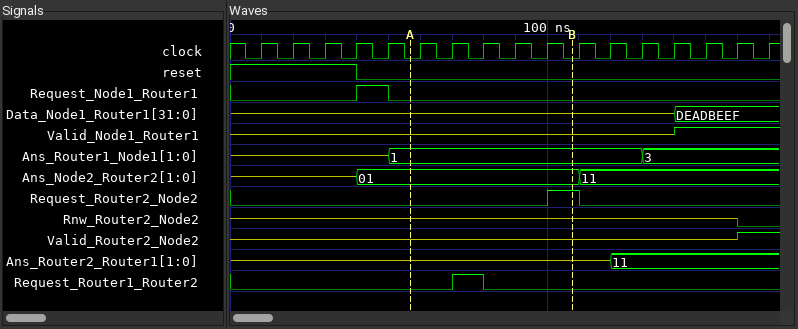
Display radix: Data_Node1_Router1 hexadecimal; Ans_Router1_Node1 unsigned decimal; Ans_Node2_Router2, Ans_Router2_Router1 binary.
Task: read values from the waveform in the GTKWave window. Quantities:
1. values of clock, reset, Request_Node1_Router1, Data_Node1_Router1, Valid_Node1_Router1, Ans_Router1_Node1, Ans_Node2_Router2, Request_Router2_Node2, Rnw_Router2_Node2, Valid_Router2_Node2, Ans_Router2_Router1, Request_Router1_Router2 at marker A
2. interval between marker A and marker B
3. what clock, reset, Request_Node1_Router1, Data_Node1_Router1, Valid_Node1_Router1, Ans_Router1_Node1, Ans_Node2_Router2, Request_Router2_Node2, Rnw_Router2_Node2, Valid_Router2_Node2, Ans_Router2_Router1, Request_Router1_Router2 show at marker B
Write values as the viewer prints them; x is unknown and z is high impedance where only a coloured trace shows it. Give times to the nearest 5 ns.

clock=0, reset=0, Request_Node1_Router1=0, Data_Node1_Router1=z, Valid_Node1_Router1=z, Ans_Router1_Node1=1, Ans_Node2_Router2=01, Request_Router2_Node2=0, Rnw_Router2_Node2=z, Valid_Router2_Node2=z, Ans_Router2_Router1=z, Request_Router1_Router2=0
50 ns
clock=0, reset=0, Request_Node1_Router1=0, Data_Node1_Router1=z, Valid_Node1_Router1=z, Ans_Router1_Node1=1, Ans_Node2_Router2=01, Request_Router2_Node2=1, Rnw_Router2_Node2=z, Valid_Router2_Node2=z, Ans_Router2_Router1=z, Request_Router1_Router2=0
